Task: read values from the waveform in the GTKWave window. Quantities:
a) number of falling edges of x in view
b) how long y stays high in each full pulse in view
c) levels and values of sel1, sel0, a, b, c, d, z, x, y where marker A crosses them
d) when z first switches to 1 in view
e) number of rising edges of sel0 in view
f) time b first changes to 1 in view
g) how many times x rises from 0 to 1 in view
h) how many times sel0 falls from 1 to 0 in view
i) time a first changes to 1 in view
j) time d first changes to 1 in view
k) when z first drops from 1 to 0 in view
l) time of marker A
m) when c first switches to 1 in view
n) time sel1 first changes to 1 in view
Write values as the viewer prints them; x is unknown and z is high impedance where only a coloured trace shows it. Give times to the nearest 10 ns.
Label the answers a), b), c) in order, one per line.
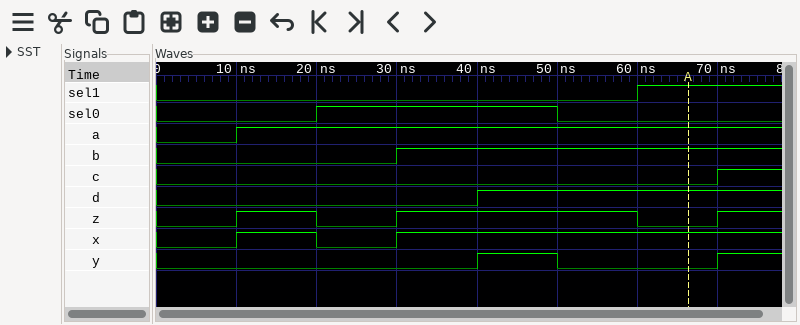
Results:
a) 1
b) 10 ns
c) sel1=1, sel0=0, a=1, b=1, c=0, d=1, z=0, x=1, y=0
d) 10 ns
e) 1
f) 30 ns
g) 2
h) 1
i) 10 ns
j) 40 ns
k) 20 ns
l) 70 ns
m) 70 ns
n) 60 ns
